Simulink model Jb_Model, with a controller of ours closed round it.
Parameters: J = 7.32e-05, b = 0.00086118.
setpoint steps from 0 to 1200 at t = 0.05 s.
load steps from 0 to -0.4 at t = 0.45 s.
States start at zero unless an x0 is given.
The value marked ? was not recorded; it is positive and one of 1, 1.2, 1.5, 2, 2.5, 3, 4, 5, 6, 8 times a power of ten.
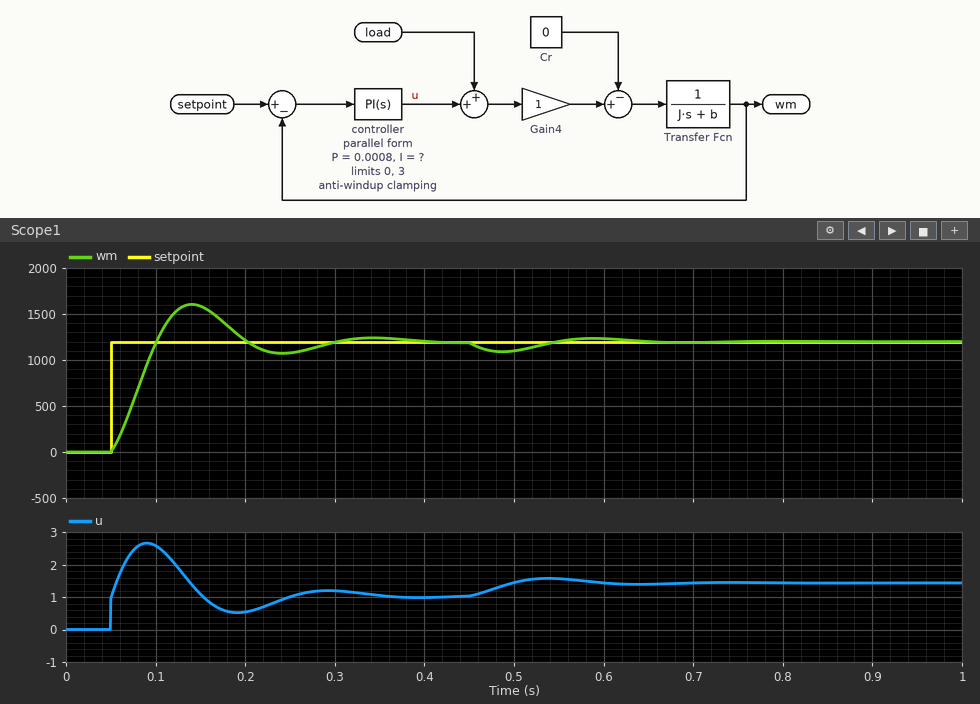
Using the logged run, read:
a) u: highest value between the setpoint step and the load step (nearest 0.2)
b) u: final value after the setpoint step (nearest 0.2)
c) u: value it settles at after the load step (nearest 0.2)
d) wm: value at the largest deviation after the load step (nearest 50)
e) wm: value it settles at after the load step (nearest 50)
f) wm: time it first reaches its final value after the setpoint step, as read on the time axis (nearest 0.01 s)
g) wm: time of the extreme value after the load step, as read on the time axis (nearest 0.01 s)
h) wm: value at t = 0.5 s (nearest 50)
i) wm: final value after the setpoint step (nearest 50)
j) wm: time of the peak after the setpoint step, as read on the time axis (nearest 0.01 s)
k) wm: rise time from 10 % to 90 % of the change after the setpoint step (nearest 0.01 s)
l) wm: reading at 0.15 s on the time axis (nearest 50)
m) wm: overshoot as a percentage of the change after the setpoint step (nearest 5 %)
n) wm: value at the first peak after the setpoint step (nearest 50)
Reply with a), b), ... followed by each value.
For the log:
a) 2.6
b) 1.0
c) 1.4
d) 1100
e) 1200
f) 0.10 s
g) 0.49 s
h) 1100
i) 1200
j) 0.14 s
k) 0.04 s
l) 1600
m) 35 %
n) 1600
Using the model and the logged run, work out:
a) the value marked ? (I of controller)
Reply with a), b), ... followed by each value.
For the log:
a) 0.08
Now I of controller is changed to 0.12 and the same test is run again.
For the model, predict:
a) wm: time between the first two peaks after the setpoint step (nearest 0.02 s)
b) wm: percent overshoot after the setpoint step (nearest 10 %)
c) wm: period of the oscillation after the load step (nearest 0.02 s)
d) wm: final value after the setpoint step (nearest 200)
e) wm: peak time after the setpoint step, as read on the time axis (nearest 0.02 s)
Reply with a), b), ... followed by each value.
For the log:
a) 0.16 s
b) 40 %
c) 0.16 s
d) 1200
e) 0.12 s
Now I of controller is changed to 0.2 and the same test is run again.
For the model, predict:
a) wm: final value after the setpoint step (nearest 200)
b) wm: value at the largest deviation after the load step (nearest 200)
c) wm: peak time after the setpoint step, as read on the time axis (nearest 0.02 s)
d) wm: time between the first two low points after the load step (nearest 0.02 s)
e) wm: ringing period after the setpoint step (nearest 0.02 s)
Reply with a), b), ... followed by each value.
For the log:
a) 1200
b) 1200
c) 0.12 s
d) 0.12 s
e) 0.12 s
